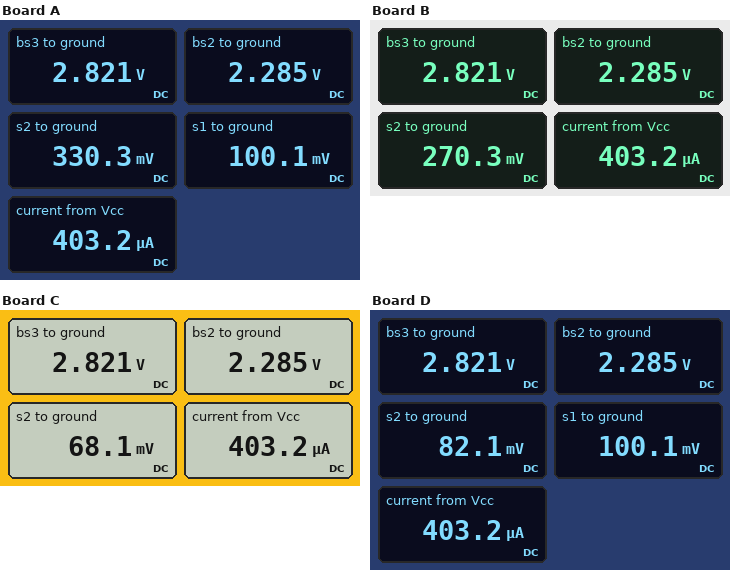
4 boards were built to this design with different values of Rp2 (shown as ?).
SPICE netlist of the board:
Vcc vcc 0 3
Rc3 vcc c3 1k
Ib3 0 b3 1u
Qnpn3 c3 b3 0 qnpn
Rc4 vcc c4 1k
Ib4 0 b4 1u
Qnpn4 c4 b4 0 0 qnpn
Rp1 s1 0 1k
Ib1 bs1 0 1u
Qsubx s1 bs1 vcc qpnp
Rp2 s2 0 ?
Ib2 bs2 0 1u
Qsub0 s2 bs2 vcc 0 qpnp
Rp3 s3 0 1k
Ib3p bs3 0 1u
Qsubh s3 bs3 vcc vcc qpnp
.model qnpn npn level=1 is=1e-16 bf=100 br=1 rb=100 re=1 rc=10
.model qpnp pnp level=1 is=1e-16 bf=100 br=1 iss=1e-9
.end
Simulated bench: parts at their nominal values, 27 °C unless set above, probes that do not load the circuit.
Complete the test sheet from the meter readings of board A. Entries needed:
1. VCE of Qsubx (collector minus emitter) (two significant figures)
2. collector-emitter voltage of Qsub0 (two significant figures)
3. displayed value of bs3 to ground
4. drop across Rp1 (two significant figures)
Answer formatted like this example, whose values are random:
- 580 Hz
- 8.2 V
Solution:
- -2.9 V
- -2.7 V
- 2.821 V
- 100 mV
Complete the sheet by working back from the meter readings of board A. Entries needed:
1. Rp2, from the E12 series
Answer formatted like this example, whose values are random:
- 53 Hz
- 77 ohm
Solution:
- 3.3 kΩ
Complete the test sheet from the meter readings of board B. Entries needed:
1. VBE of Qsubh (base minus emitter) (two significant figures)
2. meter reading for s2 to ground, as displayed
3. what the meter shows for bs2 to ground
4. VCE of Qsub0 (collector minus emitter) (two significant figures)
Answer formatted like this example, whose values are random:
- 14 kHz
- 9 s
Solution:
- -180 mV
- 270.3 mV
- 2.285 V
- -2.7 V
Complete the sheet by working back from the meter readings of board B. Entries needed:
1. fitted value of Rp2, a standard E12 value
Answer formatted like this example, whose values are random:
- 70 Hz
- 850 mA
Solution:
- 2.7 kΩ
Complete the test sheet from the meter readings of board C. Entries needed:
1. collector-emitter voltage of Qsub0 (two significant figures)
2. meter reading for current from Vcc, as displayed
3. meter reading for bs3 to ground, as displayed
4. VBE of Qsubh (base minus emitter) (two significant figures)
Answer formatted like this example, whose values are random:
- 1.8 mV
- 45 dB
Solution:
- -2.9 V
- 403.2 µA
- 2.821 V
- -180 mV
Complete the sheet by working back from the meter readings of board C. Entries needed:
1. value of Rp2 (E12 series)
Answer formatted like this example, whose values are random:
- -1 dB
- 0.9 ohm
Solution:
- 680 Ω
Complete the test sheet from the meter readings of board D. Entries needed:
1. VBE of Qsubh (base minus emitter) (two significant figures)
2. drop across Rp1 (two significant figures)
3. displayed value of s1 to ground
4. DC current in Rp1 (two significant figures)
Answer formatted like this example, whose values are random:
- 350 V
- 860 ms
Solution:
- -180 mV
- 100 mV
- 100.1 mV
- 100 µA
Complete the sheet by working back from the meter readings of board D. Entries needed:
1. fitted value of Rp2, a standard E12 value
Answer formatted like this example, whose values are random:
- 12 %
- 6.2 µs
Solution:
- 820 Ω
